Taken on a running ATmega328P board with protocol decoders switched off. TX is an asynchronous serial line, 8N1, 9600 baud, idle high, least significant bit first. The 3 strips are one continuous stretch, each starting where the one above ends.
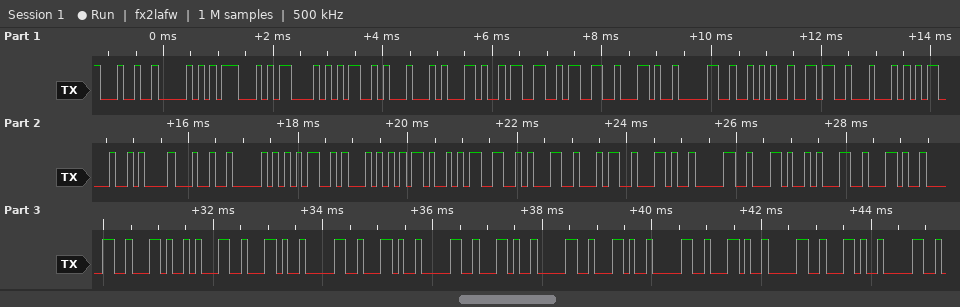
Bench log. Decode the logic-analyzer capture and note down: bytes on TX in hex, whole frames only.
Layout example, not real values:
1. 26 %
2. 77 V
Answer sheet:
1. 0x24 0x50 0x47 0x43 0x4D 0x44 0x2C 0x33 0x33 0x2C 0x30 0x2A 0x36 0x44 0x0D 0x0A 0x24 0x50 0x4D 0x54 0x4B 0x33 0x31 0x34 0x2C 0x30 0x2C 0x31 0x2C 0x30 0x2C 0x31 0x2C 0x30 0x2C 0x30 0x2C 0x30 0x2C 0x30 0x2C 0x30 0x2C 0x30
